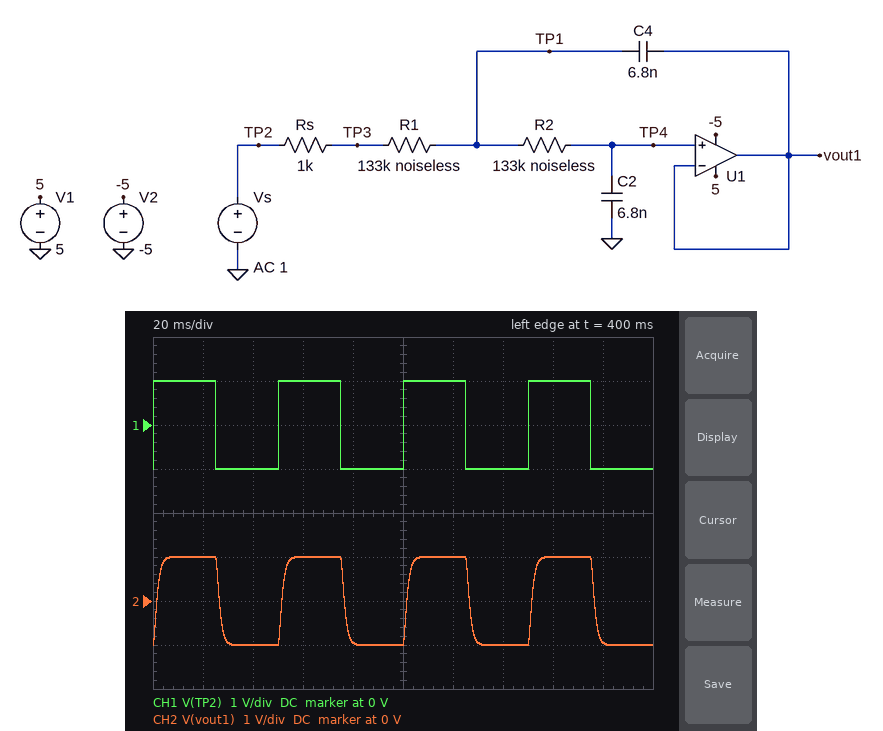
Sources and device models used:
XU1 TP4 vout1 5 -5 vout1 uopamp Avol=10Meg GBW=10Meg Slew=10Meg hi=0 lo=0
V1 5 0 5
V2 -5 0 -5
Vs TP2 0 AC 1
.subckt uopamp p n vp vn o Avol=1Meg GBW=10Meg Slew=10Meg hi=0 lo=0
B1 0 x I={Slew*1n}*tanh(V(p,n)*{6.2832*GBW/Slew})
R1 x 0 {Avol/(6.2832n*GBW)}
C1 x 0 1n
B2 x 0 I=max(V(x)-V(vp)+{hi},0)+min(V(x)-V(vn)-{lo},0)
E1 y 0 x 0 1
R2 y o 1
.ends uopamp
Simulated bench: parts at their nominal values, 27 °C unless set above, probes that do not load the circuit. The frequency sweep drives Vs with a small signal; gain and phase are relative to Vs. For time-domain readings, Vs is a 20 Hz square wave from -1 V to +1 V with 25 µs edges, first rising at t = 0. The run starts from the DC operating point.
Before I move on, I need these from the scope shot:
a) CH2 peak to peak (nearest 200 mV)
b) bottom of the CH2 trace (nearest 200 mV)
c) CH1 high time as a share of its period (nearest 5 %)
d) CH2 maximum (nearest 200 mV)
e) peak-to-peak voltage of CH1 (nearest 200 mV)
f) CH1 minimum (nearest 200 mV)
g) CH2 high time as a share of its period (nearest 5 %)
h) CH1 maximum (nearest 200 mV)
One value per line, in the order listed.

2.0 V
-1.0 V
50 %
1.0 V
2.0 V
-1.0 V
50 %
1.0 V
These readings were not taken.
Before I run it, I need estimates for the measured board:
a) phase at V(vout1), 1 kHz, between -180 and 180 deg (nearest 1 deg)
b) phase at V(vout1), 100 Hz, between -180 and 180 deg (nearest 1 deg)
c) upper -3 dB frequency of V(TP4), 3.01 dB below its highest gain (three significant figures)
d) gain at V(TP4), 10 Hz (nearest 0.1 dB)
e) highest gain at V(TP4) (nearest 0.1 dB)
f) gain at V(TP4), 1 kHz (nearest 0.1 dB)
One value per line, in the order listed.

-160 deg
-59 deg
113 Hz
0 dB
0 dB
-30.5 dB
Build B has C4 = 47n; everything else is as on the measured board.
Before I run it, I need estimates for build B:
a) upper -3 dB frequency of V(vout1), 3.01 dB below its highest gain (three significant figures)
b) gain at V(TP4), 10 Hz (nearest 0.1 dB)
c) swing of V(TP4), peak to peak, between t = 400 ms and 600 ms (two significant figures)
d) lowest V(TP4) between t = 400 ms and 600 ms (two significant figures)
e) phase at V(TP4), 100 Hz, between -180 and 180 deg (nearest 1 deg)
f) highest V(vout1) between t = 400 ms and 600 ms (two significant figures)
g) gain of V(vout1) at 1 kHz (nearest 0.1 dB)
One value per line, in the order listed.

79.3 Hz
0.1 dB
3.1 V
-1.6 V
-138 deg
1.6 V
-47.0 dB
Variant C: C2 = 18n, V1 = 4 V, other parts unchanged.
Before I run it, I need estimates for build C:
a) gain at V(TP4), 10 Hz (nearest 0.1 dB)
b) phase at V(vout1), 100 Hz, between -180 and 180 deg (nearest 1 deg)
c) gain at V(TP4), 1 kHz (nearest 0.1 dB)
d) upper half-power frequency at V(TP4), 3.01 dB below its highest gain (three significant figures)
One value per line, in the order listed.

-0.3 dB
-87 deg
-39.1 dB
36.5 Hz
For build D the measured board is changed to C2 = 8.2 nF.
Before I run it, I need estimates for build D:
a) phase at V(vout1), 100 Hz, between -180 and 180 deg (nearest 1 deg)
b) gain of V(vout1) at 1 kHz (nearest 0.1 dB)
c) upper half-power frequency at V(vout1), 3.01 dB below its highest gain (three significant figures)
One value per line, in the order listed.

-66 deg
-32.2 dB
90.1 Hz
